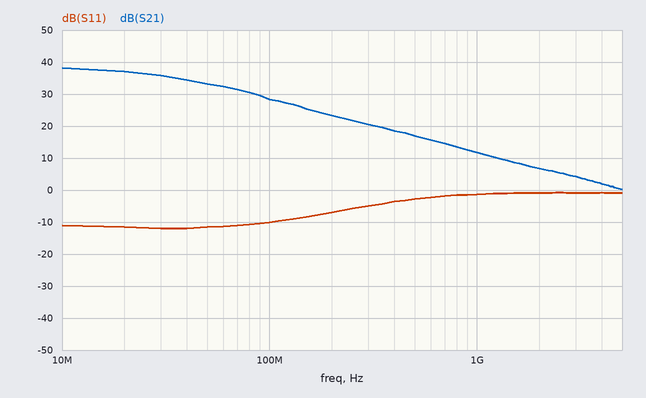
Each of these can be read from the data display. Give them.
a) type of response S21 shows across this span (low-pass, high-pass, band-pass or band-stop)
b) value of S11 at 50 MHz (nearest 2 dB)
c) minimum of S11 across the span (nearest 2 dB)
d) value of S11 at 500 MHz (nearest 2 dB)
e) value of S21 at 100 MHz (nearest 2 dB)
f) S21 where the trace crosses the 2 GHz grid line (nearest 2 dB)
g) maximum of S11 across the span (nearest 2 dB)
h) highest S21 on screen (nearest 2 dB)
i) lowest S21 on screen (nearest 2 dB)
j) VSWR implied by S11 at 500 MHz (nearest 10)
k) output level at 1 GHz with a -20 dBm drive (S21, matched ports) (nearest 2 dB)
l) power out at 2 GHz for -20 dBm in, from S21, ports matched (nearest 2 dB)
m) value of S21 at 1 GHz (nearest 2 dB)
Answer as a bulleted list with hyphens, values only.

- low-pass
- -12 dB
- -12 dB
- -2 dB
- 28 dB
- 6 dB
- 0 dB
- 38 dB
- 0 dB
- 10
- -8 dBm
- -14 dBm
- 12 dB
